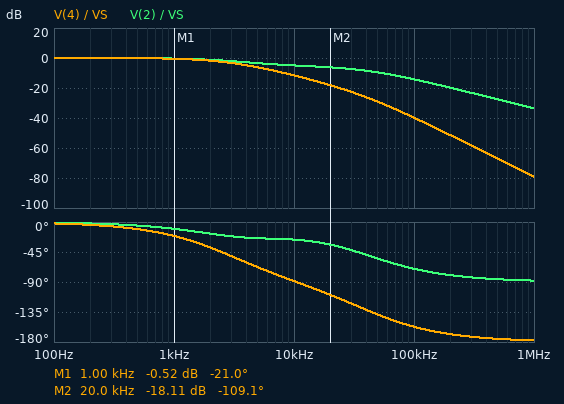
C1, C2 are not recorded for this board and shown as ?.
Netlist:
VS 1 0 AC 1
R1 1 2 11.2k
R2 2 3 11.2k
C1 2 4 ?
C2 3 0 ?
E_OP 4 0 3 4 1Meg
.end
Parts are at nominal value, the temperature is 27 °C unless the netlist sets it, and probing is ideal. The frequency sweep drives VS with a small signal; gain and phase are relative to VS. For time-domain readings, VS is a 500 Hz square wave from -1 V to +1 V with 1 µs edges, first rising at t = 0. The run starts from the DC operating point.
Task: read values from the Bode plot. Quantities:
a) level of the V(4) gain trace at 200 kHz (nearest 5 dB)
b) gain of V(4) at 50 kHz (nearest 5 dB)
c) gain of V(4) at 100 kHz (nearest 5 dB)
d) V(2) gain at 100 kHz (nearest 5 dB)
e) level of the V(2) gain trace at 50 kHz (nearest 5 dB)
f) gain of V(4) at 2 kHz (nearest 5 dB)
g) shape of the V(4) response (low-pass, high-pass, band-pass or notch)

-50 dB
-30 dB
-40 dB
-15 dB
-10 dB
0 dB
low-pass
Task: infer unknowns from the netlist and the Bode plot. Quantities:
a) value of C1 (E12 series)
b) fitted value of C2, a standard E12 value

680 pF
2.7 nF
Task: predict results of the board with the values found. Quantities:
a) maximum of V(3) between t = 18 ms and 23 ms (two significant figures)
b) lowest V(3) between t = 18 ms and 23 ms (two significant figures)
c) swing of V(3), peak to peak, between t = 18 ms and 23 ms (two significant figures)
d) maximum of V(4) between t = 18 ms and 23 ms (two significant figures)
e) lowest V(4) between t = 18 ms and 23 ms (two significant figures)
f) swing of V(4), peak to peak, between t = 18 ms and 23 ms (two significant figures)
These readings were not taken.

1.0 V
-1.0 V
2.0 V
1.0 V
-1.0 V
2.0 V
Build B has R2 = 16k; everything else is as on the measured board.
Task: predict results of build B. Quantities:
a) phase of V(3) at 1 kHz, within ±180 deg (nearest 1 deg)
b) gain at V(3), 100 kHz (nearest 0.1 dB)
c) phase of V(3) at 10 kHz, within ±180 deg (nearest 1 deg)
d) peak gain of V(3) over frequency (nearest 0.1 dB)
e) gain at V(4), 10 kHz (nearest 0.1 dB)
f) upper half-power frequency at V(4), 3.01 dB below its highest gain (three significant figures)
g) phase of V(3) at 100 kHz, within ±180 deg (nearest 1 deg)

-25 deg
-42.7 dB
-94 deg
0 dB
-13.3 dB
2.31 kHz
-160 deg
